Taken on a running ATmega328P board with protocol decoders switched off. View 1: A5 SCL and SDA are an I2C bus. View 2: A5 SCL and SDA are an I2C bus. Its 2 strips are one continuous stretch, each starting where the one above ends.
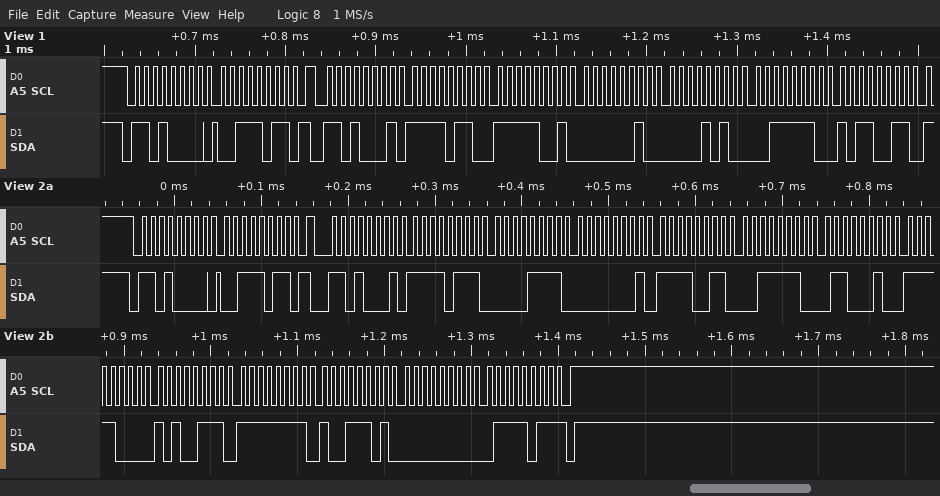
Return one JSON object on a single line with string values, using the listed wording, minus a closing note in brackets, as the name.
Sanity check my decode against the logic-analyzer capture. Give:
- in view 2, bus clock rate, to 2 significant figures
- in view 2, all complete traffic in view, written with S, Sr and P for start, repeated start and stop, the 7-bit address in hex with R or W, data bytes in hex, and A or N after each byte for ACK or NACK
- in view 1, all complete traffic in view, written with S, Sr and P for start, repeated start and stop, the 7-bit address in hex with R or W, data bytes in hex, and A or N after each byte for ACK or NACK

{"in view 2, bus clock rate, to 2 significant figures": "100 kHz", "in view 2, all complete traffic in view, written with S, Sr and P for start, repeated start and stop, the 7-bit address in hex with R or W, data bytes in hex, and A or N after each byte for ACK or NACK": "S 68W A 3B A Sr 68R A F7 A 0F A 01 A F3 A 3E A 62 A F8 A A7 A FF A 9D A 00 A 7B N P", "in view 1, all complete traffic in view, written with S, Sr and P for start, repeated start and stop, the 7-bit address in hex with R or W, data bytes in hex, and A or N after each byte for ACK or NACK": "S 68W A 3B A Sr 68R A F6 A F9 A 02 A 0A A 3E A B3 A"}
